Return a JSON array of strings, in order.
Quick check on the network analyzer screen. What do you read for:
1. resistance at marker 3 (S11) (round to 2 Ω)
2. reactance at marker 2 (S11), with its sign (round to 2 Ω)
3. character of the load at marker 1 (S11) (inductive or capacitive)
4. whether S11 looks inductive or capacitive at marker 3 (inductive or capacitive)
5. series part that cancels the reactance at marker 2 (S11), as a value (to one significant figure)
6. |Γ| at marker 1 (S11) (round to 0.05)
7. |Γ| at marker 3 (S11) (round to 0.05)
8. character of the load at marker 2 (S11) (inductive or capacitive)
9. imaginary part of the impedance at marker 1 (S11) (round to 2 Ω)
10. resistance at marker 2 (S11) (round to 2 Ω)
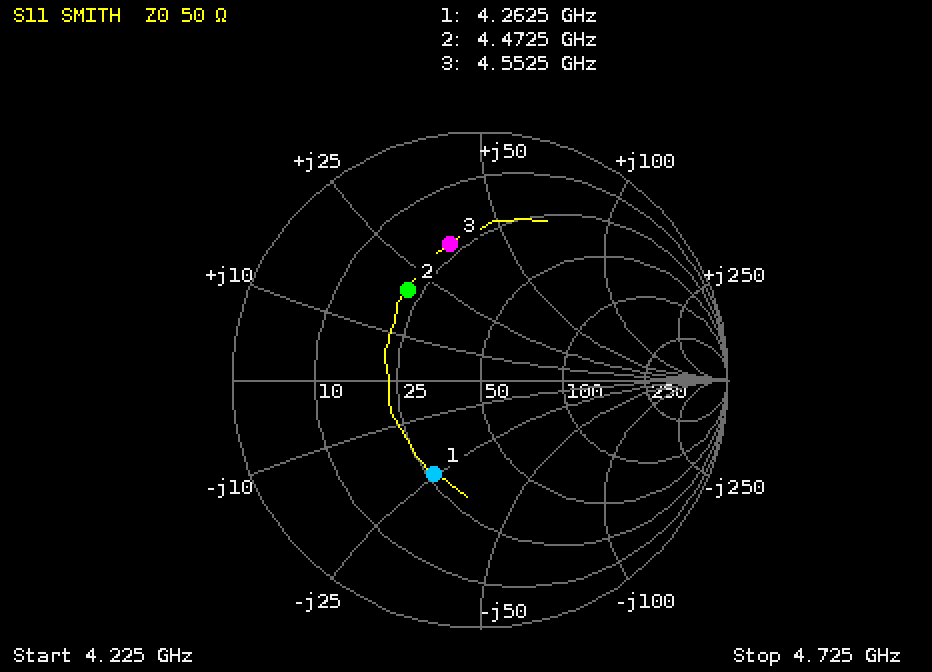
["22 Ω", "+20 Ω", "capacitive", "inductive", "2 pF", "0.40", "0.55", "inductive", "-24 Ω", "22 Ω"]
